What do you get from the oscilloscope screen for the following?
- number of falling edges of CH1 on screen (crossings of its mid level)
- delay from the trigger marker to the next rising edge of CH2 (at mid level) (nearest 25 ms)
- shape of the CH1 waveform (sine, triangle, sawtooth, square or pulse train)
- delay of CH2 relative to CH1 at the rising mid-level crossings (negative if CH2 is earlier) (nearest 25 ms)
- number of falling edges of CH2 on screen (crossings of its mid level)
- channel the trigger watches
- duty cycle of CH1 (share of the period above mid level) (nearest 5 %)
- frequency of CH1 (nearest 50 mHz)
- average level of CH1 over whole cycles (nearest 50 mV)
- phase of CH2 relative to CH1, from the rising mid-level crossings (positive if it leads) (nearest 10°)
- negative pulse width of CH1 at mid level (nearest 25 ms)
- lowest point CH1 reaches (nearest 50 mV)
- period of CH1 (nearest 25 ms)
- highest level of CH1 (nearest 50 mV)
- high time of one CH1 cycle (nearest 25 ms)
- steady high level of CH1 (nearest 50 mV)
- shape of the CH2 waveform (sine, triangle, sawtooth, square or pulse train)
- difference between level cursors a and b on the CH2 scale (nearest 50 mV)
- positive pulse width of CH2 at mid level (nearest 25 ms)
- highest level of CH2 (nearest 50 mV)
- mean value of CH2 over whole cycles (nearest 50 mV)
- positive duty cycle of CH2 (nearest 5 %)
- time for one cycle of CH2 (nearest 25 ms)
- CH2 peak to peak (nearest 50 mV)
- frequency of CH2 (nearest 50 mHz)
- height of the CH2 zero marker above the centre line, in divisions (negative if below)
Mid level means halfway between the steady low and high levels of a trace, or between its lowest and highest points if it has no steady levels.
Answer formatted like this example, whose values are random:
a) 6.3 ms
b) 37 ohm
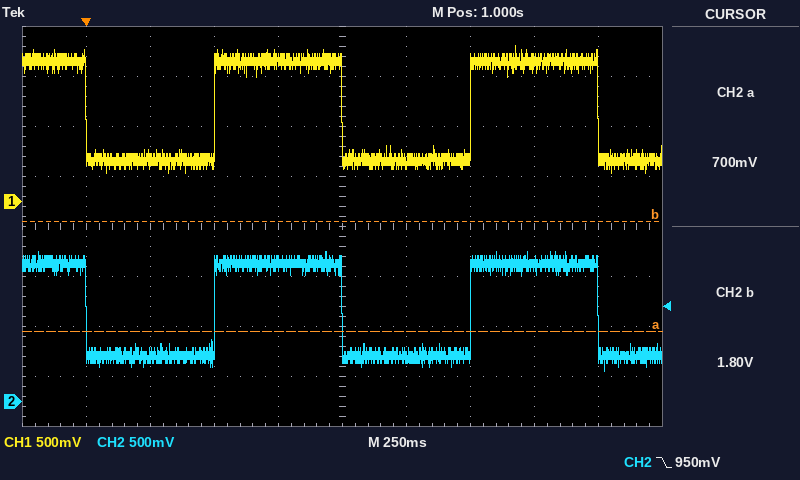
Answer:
a) 3
b) 500 ms
c) square
d) 0 ms
e) 3
f) CH2
g) 50 %
h) 1.00 Hz
i) 900 mV
j) 0°
k) 500 ms
l) 300 mV
m) 1.000 s
n) 1.55 V
o) 500 ms
p) 1.40 V
q) square
r) 1.10 V
s) 500 ms
t) 1.50 V
u) 900 mV
v) 50 %
w) 1.000 s
x) 1.20 V
y) 1.00 Hz
z) -3.5 div
